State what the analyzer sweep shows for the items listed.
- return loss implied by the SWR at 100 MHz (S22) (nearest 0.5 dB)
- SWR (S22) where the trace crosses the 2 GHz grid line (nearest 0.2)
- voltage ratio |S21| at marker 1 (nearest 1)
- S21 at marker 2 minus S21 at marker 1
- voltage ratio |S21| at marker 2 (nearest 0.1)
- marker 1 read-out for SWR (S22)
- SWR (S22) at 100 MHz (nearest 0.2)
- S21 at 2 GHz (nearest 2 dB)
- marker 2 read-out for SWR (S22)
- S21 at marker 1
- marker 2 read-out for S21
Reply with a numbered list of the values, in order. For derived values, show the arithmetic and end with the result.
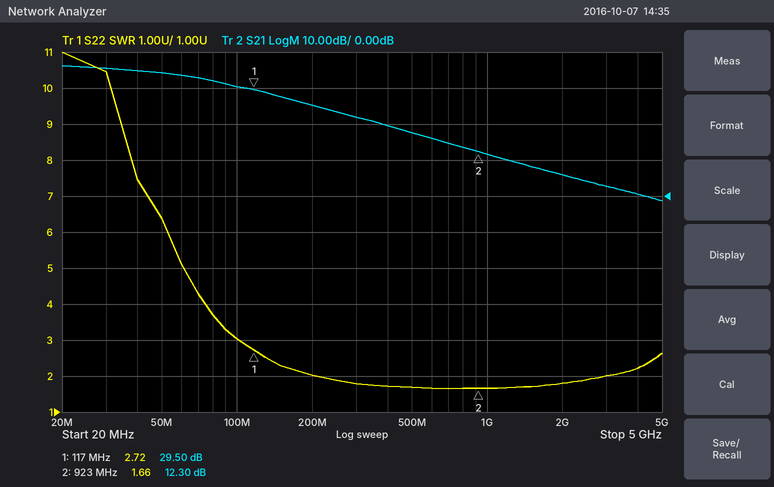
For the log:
1. −20 log10((3 − 1)/(3 + 1)) ≈ 6.0 dB
2. 1.8
3. 10^(29.5/20) ≈ 30
4. 12.3 − (29.5) = -17.20 dB
5. 10^(12.3/20) ≈ 4.1
6. 2.72
7. 3.0
8. 6 dB
9. 1.66
10. 29.50 dB
11. 12.30 dB
